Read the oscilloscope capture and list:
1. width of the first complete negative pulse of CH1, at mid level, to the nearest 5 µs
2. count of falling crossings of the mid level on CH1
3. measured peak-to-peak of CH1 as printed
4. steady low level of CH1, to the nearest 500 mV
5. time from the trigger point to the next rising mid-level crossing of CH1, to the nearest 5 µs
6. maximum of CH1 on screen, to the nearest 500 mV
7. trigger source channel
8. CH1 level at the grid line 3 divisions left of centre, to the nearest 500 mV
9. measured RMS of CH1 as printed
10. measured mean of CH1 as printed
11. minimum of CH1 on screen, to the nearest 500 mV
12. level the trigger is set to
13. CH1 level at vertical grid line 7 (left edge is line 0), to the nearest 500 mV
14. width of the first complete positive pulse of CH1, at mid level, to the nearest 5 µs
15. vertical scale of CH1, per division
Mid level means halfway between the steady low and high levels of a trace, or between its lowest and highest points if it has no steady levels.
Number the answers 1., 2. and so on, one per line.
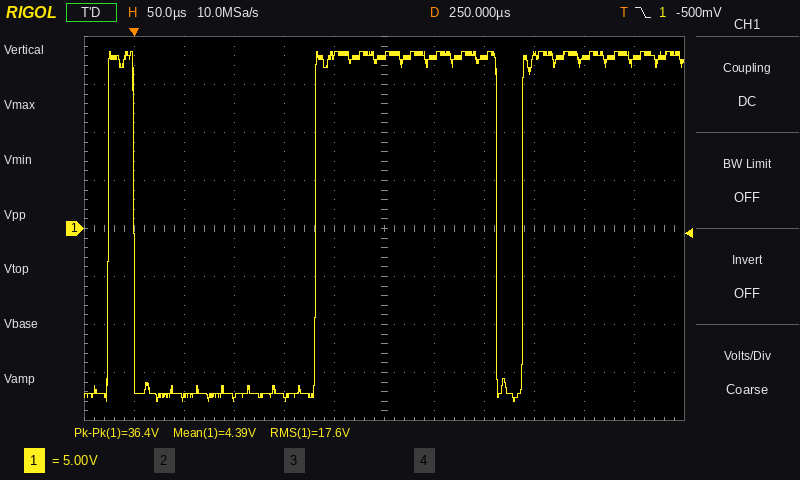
1. 180 µs
2. 2
3. 36.4 V
4. -17.0 V
5. 180 µs
6. 18.5 V
7. CH1
8. -17.5 V
9. 17.6 V
10. 4.39 V
11. -18.0 V
12. -500 mV
13. 18.0 V
14. 25 µs
15. 5 V
